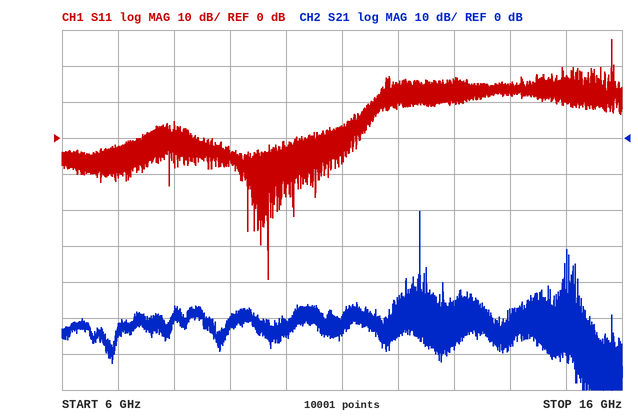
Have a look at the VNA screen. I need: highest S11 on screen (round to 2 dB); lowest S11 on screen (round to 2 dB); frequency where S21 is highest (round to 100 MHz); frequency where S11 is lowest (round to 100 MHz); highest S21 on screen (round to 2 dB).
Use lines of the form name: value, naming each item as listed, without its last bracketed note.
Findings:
highest S11 on screen: 28 dB
lowest S11 on screen: -40 dB
frequency where S21 is highest: 12.4 GHz
frequency where S11 is lowest: 9.7 GHz
highest S21 on screen: -20 dB
